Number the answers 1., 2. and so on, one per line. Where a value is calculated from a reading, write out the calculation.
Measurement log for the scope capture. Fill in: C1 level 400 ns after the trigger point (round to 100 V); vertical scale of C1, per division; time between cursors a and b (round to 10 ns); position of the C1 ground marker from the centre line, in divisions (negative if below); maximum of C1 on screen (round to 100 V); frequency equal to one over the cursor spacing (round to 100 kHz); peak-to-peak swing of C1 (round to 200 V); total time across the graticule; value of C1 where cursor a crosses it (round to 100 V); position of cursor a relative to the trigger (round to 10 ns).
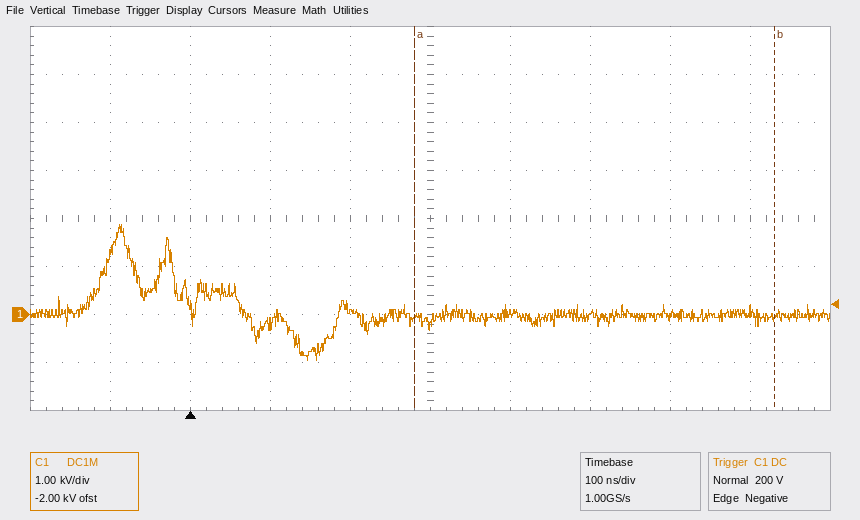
1. 0.0 kV
2. 1 kV
3. 450 ns
4. -2.0 div
5. 1.9 kV
6. 1 / 450 ns ≈ 2.2 MHz
7. 2.8 kV
8. 1 µs
9. -100 V
10. +280 ns
